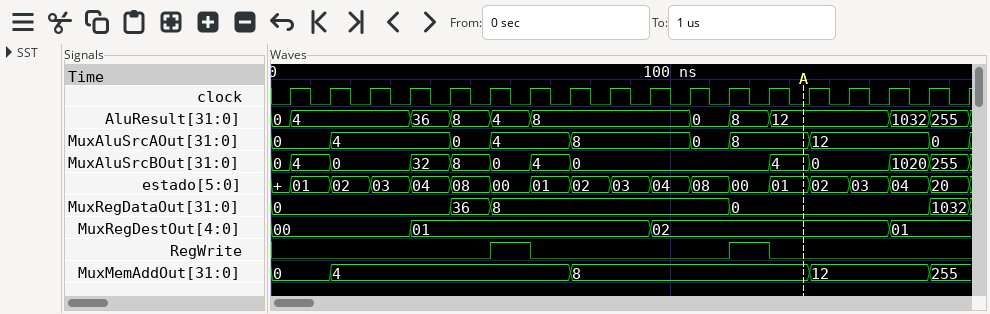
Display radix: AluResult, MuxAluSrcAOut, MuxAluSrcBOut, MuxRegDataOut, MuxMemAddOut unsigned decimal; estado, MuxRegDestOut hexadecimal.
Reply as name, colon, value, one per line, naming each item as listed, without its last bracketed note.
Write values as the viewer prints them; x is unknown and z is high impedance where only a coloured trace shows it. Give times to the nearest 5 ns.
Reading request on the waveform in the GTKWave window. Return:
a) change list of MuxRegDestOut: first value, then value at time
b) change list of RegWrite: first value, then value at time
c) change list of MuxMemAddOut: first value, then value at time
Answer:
change list of MuxRegDestOut: first value, then value at time: 00, 01 at 35 ns, 02 at 95 ns, 01 at 155 ns
change list of RegWrite: first value, then value at time: 0, 1 at 55 ns, 0 at 65 ns, 1 at 115 ns, 0 at 125 ns
change list of MuxMemAddOut: first value, then value at time: 0, 4 at 15 ns, 8 at 75 ns, 12 at 135 ns, 255 at 165 ns
